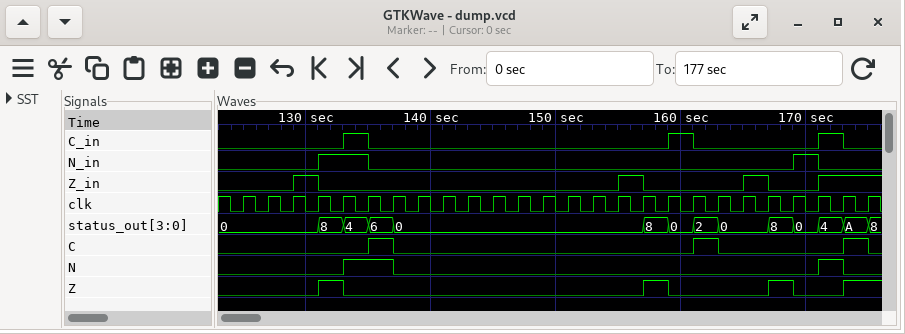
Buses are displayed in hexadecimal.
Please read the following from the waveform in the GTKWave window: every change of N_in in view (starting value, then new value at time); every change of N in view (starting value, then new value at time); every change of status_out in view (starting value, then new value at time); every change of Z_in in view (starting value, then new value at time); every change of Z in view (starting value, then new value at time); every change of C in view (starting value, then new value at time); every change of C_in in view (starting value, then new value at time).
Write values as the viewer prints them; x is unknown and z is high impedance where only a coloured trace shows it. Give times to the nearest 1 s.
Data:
0, 1 at 131 s, 0 at 135 s, 1 at 169 s, 0 at 171 s
0, 1 at 133 s, 0 at 137 s, 1 at 171 s, 0 at 173 s
0, 8 at 131 s, 4 at 133 s, 6 at 135 s, 0 at 137 s, 8 at 157 s, 0 at 159 s, 2 at 161 s, 0 at 163 s, 8 at 167 s, 0 at 169 s, 4 at 171 s, A at 173 s, 8 at 175 s
0, 1 at 129 s, 0 at 131 s, 1 at 155 s, 0 at 157 s, 1 at 165 s, 0 at 167 s, 1 at 171 s
0, 1 at 131 s, 0 at 133 s, 1 at 157 s, 0 at 159 s, 1 at 167 s, 0 at 169 s, 1 at 173 s
0, 1 at 135 s, 0 at 137 s, 1 at 161 s, 0 at 163 s, 1 at 173 s, 0 at 175 s
0, 1 at 133 s, 0 at 135 s, 1 at 159 s, 0 at 161 s, 1 at 171 s, 0 at 173 s
